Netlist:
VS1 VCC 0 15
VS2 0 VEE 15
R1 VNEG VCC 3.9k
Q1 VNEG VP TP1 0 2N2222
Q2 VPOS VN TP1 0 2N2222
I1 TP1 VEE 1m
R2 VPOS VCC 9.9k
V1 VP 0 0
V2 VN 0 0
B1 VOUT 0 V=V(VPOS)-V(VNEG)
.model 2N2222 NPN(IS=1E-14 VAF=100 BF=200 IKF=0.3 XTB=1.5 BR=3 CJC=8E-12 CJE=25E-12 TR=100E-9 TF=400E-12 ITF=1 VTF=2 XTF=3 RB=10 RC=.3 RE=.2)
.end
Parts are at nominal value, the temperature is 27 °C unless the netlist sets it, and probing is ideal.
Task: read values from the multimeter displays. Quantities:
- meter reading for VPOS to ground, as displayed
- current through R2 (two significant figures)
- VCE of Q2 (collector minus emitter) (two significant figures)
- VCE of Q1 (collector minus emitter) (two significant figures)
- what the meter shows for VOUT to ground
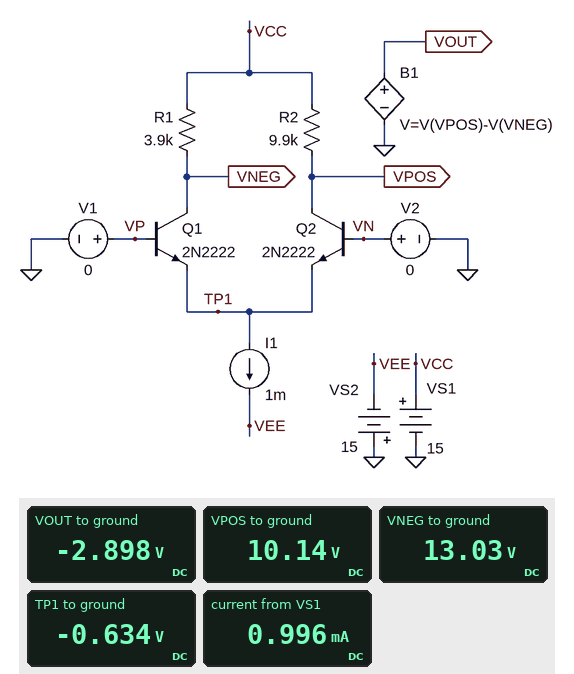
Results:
10.14 V
490 µA
11 V
14 V
-2.898 V
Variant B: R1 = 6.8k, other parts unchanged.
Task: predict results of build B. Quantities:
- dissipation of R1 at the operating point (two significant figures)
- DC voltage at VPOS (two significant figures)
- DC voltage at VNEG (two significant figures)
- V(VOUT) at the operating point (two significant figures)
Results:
1.7 mW
10 V
12 V
-1.5 V
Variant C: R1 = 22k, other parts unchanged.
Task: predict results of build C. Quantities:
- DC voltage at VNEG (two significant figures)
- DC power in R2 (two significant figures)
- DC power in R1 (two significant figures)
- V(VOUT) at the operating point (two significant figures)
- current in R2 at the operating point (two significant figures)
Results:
4.3 V
2.6 mW
5.2 mW
5.6 V
510 µA
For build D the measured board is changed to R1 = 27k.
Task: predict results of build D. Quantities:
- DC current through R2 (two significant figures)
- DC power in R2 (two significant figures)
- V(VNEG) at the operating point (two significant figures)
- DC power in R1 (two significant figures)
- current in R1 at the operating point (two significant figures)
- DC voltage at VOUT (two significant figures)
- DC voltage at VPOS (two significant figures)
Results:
520 µA
2.6 mW
2.1 V
6.2 mW
480 µA
7.8 V
9.9 V
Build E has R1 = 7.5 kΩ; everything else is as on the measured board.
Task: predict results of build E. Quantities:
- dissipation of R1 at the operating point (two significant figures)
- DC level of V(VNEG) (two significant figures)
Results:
1.9 mW
11 V
